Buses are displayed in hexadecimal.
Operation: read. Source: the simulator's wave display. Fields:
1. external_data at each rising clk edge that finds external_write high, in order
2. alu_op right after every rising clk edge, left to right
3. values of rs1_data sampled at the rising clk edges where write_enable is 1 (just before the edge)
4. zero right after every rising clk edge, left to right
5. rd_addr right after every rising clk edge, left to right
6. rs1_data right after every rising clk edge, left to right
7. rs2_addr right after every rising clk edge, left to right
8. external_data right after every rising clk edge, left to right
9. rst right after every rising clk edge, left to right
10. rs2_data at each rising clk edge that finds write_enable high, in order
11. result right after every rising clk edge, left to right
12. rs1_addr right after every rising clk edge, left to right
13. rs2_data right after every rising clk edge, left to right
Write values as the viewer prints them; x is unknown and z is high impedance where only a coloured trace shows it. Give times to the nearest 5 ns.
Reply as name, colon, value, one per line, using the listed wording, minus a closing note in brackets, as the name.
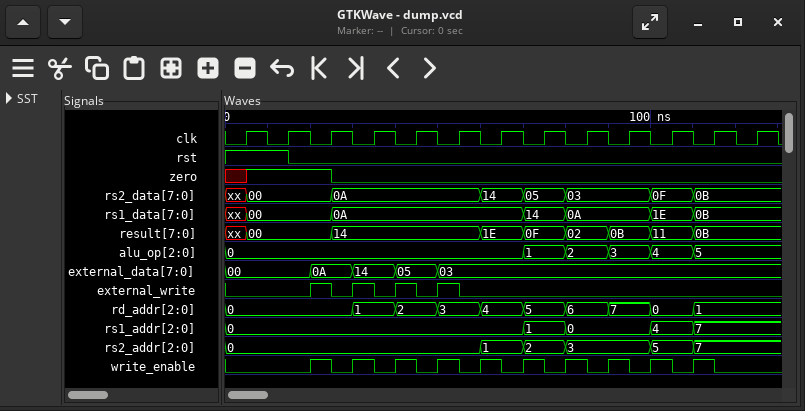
external_data at each rising clk edge that finds external_write high, in order: 0A, 14, 05, 03
alu_op right after every rising clk edge, left to right: 0, 0, 0, 0, 0, 0, 0, 1, 2, 3, 4, 5, 5
values of rs1_data sampled at the rising clk edges where write_enable is 1: 00, 0A, 0A, 0A, 0A, 14, 0A, 0A, 1E, 0B
zero right after every rising clk edge, left to right: 1 1 0 0 0 0 0 0 0 0 0 0 0
rd_addr right after every rising clk edge, left to right: 0, 0, 0, 1, 2, 3, 4, 5, 6, 7, 0, 1, 1
rs1_data right after every rising clk edge, left to right: 00, 00, 0A, 0A, 0A, 0A, 0A, 14, 0A, 0A, 1E, 0B, 0B
rs2_addr right after every rising clk edge, left to right: 0, 0, 0, 0, 0, 0, 1, 2, 3, 3, 5, 7, 7
external_data right after every rising clk edge, left to right: 00, 00, 0A, 14, 05, 03, 03, 03, 03, 03, 03, 03, 03
rst right after every rising clk edge, left to right: 1 0 0 0 0 0 0 0 0 0 0 0 0
rs2_data at each rising clk edge that finds write_enable high, in order: 00, 0A, 0A, 0A, 14, 05, 03, 03, 0F, 0B
result right after every rising clk edge, left to right: 00, 00, 14, 14, 14, 14, 1E, 0F, 02, 0B, 11, 0B, 0B
rs1_addr right after every rising clk edge, left to right: 0, 0, 0, 0, 0, 0, 0, 1, 0, 0, 4, 7, 7
rs2_data right after every rising clk edge, left to right: 00, 00, 0A, 0A, 0A, 0A, 14, 05, 03, 03, 0F, 0B, 0B
